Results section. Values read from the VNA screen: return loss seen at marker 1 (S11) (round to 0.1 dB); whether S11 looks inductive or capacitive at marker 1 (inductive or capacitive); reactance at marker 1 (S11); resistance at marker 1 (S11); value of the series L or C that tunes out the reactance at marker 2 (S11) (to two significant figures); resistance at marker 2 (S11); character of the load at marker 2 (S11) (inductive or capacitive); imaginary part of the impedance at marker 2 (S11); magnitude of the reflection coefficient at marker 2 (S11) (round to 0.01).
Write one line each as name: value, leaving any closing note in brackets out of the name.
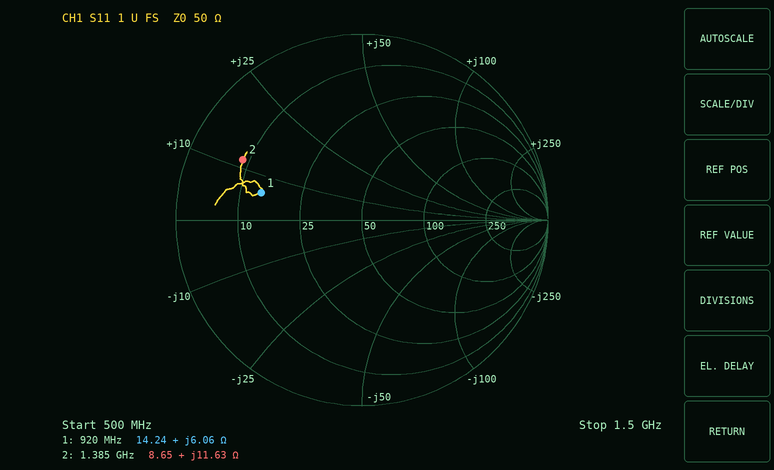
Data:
return loss seen at marker 1 (S11): 5.0 dB
whether S11 looks inductive or capacitive at marker 1: inductive
reactance at marker 1: +6.06 Ω
resistance at marker 1: 14.24 Ω
value of the series L or C that tunes out the reactance at marker 2 (S11): 9.9 pF
resistance at marker 2: 8.65 Ω
character of the load at marker 2 (S11): inductive
imaginary part of the impedance at marker 2: +11.63 Ω
magnitude of the reflection coefficient at marker 2 (S11): 0.72
